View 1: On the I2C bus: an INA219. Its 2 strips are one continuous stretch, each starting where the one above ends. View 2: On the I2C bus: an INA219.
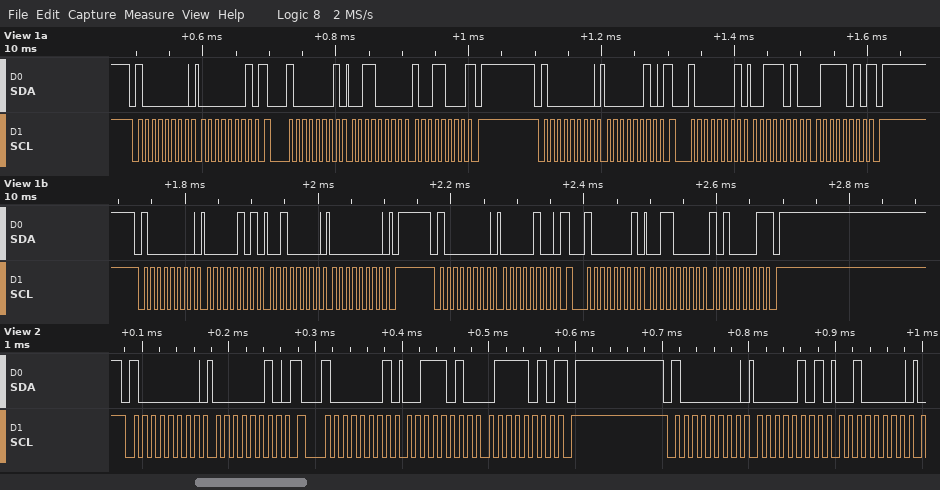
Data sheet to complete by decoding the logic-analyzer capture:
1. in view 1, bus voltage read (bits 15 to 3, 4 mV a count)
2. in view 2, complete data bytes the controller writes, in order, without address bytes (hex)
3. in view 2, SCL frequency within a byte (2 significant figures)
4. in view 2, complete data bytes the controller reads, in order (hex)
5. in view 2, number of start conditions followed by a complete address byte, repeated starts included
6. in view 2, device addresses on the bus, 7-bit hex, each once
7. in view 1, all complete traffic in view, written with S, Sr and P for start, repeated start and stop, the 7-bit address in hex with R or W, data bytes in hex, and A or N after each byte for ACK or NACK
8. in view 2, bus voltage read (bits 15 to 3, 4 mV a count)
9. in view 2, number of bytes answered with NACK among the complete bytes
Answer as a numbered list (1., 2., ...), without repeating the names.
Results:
1. 7.484 V
2. 02 05 20
3. 100 kHz
4. 3A 7A
5. 3
6. 0x40
7. S 40W A 01 A Sr 40R A 30 A 98 N P S 40W A 02 A Sr 40R A 3A A 7A N P S 40W A 05 A 20 A 00 A P S 40W A 04 A Sr 40R A 30 A A1 N P
8. 7.484 V
9. 1
